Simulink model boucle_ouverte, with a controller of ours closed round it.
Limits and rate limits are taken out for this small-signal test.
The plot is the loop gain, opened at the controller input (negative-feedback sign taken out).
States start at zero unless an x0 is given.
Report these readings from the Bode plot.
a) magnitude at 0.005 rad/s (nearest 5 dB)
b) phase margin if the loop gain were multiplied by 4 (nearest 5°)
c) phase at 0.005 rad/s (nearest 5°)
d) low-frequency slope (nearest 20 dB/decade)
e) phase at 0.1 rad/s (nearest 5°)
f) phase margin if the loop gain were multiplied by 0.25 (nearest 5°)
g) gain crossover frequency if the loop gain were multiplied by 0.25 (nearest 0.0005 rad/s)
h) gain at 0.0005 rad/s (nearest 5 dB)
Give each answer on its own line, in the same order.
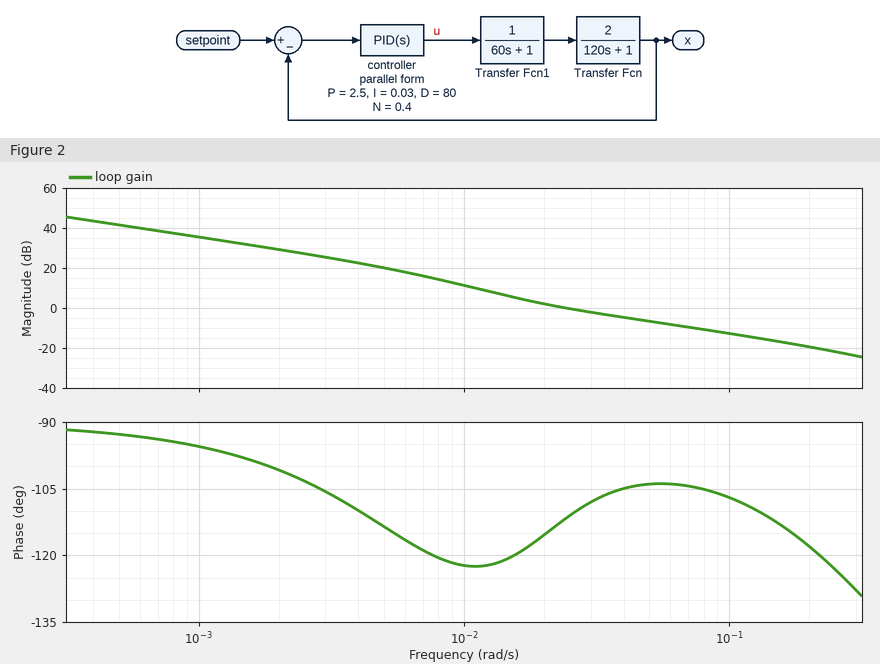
20 dB
75°
-115°
-20 dB/decade
-105°
60°
0.0095 rad/s
40 dB
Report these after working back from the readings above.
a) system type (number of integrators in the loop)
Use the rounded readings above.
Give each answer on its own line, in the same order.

1
